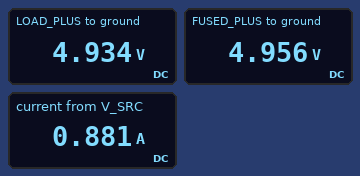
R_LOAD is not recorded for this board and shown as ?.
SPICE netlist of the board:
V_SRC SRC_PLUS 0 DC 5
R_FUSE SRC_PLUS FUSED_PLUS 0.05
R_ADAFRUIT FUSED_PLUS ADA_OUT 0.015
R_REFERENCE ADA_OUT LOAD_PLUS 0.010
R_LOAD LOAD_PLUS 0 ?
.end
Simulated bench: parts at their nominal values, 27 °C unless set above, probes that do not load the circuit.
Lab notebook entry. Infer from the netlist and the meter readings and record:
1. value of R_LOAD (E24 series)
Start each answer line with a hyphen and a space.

- 5.6 Ω
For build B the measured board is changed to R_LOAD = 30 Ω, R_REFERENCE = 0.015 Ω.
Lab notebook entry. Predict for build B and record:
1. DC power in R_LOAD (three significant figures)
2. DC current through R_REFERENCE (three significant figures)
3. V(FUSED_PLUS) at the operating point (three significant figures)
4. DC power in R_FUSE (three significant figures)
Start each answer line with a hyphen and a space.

- 829 mW
- 166 mA
- 4.99 V
- 1.38 mW
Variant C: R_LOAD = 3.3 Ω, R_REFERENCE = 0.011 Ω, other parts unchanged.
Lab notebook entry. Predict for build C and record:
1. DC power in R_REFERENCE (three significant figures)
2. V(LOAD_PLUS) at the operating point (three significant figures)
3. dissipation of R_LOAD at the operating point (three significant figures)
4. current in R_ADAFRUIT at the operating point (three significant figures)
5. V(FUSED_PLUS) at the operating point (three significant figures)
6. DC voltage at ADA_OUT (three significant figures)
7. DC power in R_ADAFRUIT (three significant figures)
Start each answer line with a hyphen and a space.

- 24.1 mW
- 4.89 V
- 7.24 W
- 1.48 A
- 4.93 V
- 4.90 V
- 32.9 mW
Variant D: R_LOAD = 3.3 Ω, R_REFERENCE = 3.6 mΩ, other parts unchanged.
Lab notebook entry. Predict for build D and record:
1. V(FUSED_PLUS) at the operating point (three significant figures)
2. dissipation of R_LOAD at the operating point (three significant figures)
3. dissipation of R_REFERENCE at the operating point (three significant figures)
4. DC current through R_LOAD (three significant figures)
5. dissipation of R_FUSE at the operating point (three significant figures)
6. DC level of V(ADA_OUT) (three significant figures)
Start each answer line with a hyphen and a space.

- 4.93 V
- 7.27 W
- 7.93 mW
- 1.48 A
- 110 mW
- 4.90 V
